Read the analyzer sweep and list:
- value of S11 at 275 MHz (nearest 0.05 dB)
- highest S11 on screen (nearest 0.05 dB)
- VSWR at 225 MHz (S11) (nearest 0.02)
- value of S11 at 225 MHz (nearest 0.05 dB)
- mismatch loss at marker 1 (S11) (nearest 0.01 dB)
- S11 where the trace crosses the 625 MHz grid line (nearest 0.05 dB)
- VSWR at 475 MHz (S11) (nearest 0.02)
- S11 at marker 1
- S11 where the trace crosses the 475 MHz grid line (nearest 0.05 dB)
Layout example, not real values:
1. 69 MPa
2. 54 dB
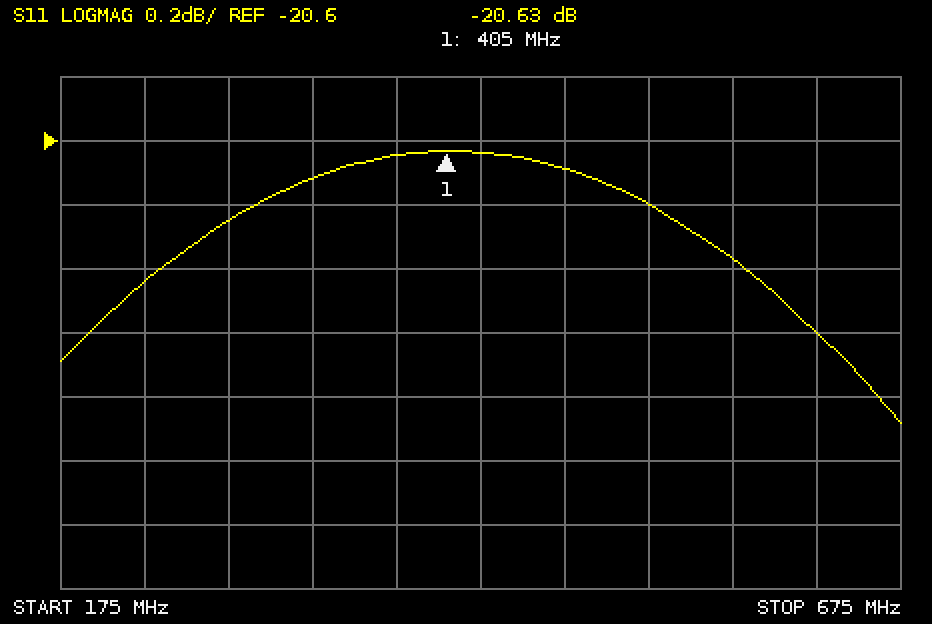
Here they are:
1. -20.85 dB
2. -20.65 dB
3. 1.20
4. -21.05 dB
5. 0.04 dB
6. -21.20 dB
7. 1.20
8. -20.63 dB
9. -20.70 dB
